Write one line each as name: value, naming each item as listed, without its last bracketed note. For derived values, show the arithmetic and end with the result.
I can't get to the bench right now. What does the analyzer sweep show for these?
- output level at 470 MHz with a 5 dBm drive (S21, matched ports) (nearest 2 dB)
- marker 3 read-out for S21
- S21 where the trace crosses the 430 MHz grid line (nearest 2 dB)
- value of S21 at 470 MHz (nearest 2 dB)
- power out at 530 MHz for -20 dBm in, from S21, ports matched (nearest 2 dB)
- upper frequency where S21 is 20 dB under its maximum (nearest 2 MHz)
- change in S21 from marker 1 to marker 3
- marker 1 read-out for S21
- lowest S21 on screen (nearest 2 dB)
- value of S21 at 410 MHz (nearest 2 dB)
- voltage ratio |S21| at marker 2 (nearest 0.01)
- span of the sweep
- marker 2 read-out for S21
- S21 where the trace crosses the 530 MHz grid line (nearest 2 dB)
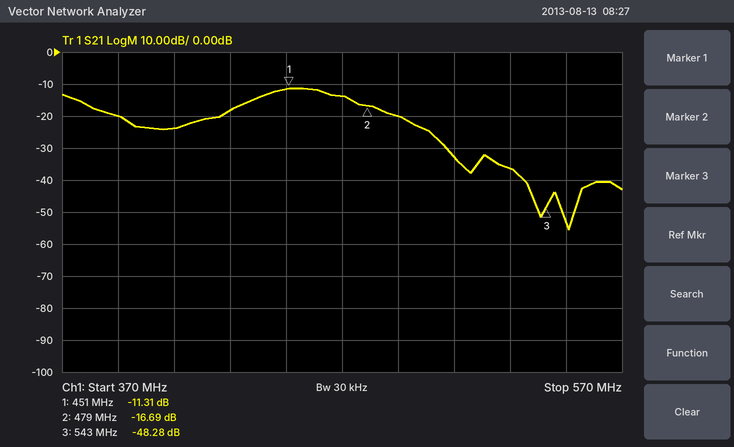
output level at 470 MHz with a 5 dBm drive (S21, matched ports): 5 dBm + (-14 dB) = -8 dBm
marker 3 read-out for S21: -48.28 dB
S21 where the trace crosses the 430 MHz grid line: -18 dB
value of S21 at 470 MHz: -14 dB
power out at 530 MHz for -20 dBm in, from S21, ports matched: -20 dBm + (-36 dB) = -56 dBm
upper frequency where S21 is 20 dB under its maximum: 508 MHz
change in S21 from marker 1 to marker 3: -48.28 − (-11.31) = -36.97 dB
marker 1 read-out for S21: -11.31 dB
lowest S21 on screen: -56 dB
value of S21 at 410 MHz: -24 dB
voltage ratio |S21| at marker 2: 10^(-16.69/20) ≈ 0.15
span of the sweep: 200 MHz
marker 2 read-out for S21: -16.69 dB
S21 where the trace crosses the 530 MHz grid line: -36 dB
